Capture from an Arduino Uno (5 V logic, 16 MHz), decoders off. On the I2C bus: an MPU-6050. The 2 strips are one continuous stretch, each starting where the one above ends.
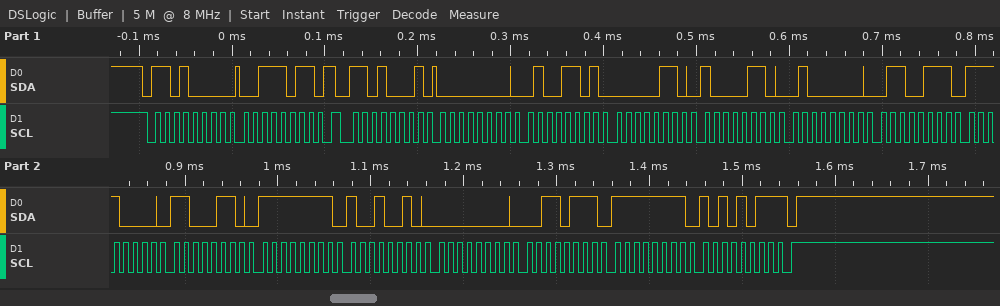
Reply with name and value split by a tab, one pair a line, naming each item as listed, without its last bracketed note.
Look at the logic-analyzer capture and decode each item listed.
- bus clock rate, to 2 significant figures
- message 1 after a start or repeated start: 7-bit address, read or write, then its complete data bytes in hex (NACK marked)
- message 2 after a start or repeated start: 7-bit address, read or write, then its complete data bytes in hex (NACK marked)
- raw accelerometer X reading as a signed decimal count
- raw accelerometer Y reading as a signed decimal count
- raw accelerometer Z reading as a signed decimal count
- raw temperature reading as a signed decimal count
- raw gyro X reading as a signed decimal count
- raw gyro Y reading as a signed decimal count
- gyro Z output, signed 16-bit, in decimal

bus clock rate, to 2 significant figures	100 kHz
message 1 after a start or repeated start: 7-bit address, read or write, then its complete data bytes in hex	0x68 write: 3B
message 2 after a start or repeated start: 7-bit address, read or write, then its complete data bytes in hex	0x68 read: 00 4D 06 86 40 67 F0 C6 FF 92 00 37 FF AB NACK
raw accelerometer X reading as a signed decimal count	77
raw accelerometer Y reading as a signed decimal count	1670
raw accelerometer Z reading as a signed decimal count	16487
raw temperature reading as a signed decimal count	-3898
raw gyro X reading as a signed decimal count	-110
raw gyro Y reading as a signed decimal count	55
gyro Z output, signed 16-bit, in decimal	-85
